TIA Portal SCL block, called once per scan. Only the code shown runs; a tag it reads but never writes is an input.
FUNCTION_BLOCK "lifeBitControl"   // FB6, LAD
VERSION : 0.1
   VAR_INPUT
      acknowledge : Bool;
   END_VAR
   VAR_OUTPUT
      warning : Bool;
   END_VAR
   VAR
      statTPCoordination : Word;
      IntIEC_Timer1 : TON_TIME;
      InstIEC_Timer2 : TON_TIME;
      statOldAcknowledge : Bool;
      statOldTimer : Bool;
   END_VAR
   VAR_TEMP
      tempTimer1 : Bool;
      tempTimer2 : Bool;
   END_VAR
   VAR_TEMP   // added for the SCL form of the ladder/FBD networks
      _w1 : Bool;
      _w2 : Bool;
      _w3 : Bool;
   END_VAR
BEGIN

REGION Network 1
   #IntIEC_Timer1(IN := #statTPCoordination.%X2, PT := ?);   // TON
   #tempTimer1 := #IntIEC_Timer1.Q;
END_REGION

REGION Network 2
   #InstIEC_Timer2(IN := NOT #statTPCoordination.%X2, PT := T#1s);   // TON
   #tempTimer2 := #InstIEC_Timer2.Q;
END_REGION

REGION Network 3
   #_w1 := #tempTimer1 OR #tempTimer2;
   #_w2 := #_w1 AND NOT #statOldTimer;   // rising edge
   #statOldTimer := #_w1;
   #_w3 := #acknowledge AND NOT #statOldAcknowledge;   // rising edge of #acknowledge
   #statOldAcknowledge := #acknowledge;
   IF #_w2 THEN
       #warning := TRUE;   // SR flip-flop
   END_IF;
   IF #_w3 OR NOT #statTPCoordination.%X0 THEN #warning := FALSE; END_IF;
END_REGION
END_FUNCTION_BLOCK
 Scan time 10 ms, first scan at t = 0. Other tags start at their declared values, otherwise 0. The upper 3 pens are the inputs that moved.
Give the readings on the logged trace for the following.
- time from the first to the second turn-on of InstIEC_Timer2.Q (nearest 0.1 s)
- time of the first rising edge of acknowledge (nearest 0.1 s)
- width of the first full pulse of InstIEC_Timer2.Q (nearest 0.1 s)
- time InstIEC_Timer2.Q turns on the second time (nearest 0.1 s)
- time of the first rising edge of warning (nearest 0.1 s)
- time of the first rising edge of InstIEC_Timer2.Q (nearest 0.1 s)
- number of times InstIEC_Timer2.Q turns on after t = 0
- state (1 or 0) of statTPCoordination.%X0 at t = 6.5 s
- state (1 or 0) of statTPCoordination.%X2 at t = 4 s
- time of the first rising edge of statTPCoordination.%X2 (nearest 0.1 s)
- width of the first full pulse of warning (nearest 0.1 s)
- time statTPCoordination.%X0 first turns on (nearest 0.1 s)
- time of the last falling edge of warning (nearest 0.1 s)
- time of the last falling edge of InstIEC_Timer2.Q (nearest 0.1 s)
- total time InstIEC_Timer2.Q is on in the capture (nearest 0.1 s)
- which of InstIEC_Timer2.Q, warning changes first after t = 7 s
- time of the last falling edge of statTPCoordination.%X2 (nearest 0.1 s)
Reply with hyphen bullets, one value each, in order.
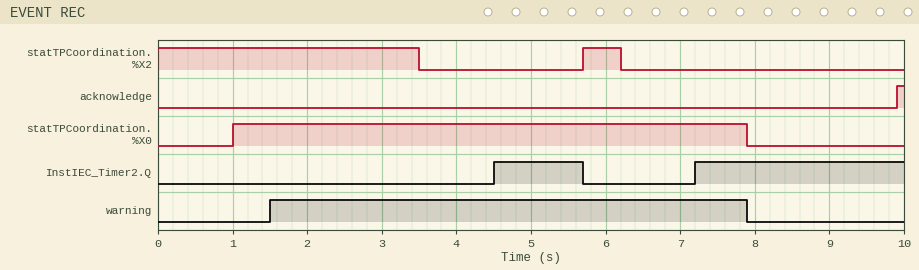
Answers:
- 2.7 s
- 9.9 s
- 1.2 s
- 7.2 s
- 1.5 s
- 4.5 s
- 2
- 1
- 0
- 5.7 s
- 6.4 s
- 1.0 s
- 7.9 s
- 5.7 s
- 4.0 s
- InstIEC_Timer2.Q
- 6.2 s
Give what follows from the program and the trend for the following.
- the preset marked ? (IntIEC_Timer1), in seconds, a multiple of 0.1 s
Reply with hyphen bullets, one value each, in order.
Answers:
- 1.5 s
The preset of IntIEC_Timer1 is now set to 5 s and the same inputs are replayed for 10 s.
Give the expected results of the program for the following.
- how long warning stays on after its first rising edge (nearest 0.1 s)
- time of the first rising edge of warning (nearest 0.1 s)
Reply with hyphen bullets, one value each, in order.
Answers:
- 3.4 s
- 4.5 s
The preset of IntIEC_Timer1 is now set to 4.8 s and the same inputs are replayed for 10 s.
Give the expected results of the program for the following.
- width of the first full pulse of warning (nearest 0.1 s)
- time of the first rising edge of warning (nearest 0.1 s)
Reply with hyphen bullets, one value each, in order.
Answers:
- 3.4 s
- 4.5 s
